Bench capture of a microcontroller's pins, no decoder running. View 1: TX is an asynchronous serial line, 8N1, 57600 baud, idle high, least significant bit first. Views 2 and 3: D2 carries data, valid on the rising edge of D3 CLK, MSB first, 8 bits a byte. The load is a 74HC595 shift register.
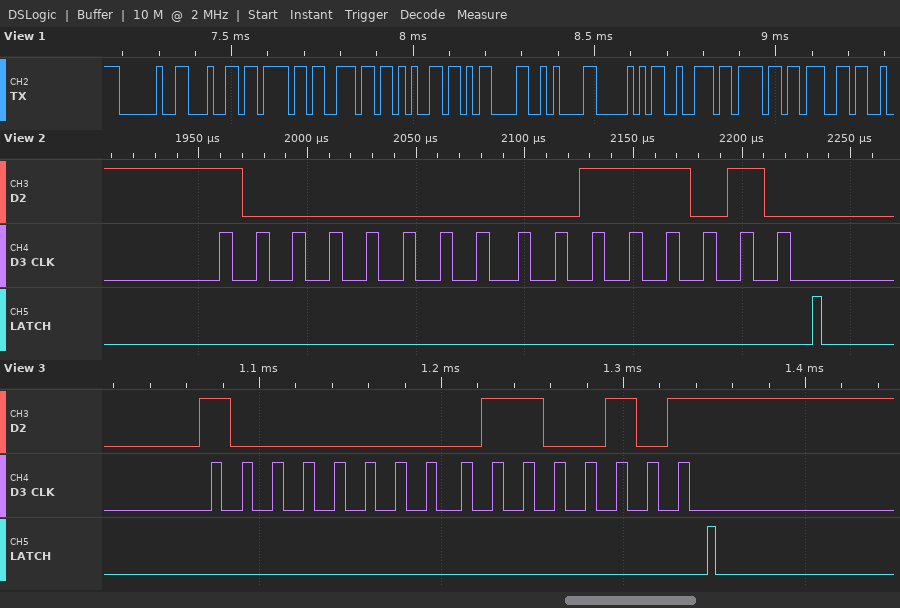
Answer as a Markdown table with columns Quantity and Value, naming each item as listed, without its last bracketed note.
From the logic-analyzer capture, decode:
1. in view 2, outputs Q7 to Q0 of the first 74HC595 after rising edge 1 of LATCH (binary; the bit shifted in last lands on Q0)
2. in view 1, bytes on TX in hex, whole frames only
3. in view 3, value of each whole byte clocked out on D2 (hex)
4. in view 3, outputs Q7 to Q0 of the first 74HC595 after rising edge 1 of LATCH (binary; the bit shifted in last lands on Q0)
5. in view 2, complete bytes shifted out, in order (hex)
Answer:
| Quantity | Value |
|---|---|
| in view 2, outputs Q7 to Q0 of the first 74HC595 after rising edge 1 of LATCH | 00111010 |
| in view 1, bytes on TX in hex, whole frames only | 20 64 6F 6E 65 0D 0A 50 72 6F 67 |
| in view 3, value of each whole byte clocked out on D2 | 0x80 0x65 |
| in view 3, outputs Q7 to Q0 of the first 74HC595 after rising edge 1 of LATCH | 01100101 |
| in view 2, complete bytes shifted out, in order | 80 3A |
